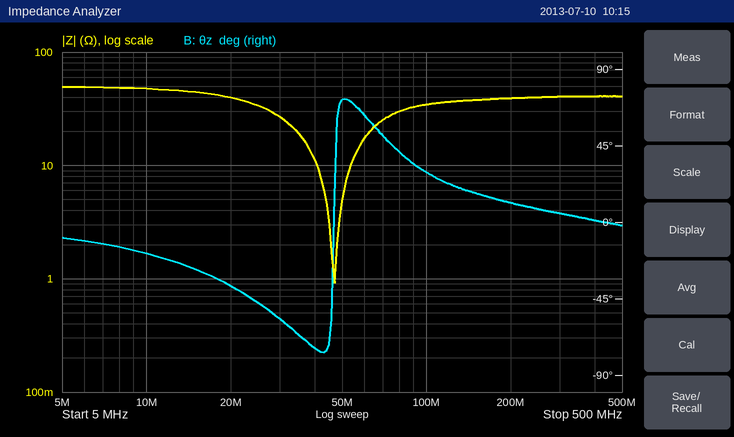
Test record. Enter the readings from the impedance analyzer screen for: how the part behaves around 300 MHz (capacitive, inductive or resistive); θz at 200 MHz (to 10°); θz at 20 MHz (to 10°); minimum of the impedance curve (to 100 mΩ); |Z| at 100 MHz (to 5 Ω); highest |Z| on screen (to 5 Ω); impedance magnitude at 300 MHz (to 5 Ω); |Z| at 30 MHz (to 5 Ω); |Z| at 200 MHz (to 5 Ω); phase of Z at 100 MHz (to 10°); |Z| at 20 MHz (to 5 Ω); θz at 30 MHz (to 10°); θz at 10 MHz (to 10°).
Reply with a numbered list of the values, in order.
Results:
1. resistive
2. 10°
3. -40°
4. 900 mΩ
5. 35 Ω
6. 50 Ω
7. 40 Ω
8. 25 Ω
9. 40 Ω
10. 30°
11. 40 Ω
12. -60°
13. -20°
